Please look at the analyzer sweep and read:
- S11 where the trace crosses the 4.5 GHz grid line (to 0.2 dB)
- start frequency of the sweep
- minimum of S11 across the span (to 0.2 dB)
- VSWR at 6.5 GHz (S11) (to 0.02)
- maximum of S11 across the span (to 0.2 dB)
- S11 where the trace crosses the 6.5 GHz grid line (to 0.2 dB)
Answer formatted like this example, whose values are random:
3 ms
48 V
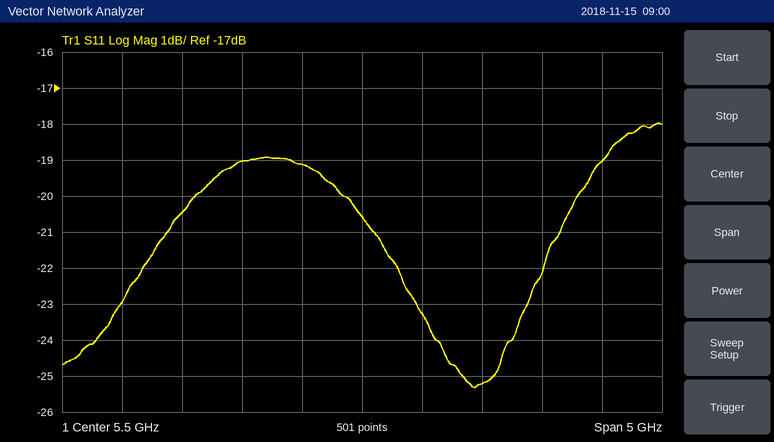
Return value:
-19.0 dB
3 GHz
-25.4 dB
1.12
-18.0 dB
-25.2 dB
